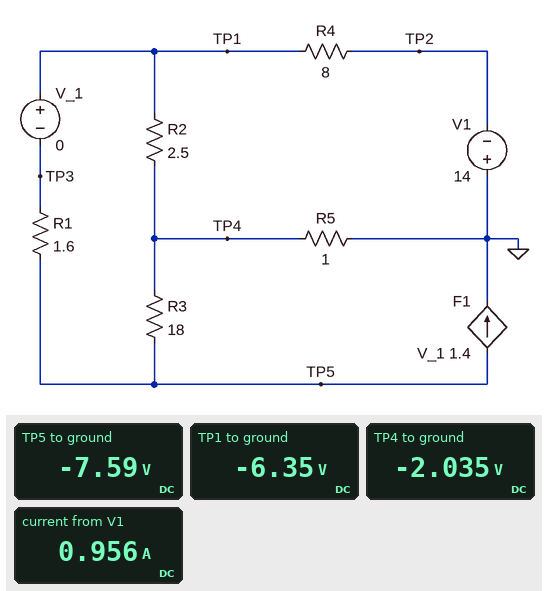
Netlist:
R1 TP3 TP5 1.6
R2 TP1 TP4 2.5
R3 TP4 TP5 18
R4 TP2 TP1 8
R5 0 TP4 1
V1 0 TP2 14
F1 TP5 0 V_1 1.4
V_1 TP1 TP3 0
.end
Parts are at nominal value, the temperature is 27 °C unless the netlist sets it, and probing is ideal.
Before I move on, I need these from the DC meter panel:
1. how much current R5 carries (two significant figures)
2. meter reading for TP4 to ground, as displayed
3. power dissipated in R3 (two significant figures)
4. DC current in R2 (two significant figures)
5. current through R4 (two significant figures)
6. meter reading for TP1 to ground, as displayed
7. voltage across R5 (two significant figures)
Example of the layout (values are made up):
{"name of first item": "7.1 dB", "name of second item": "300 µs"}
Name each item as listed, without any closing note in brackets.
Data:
{"how much current R5 carries": "2.0 A", "meter reading for TP4 to ground, as displayed": "-2.035 V", "power dissipated in R3": "1.7 W", "DC current in R2": "1.7 A", "current through R4": "960 mA", "meter reading for TP1 to ground, as displayed": "-6.35 V", "voltage across R5": "2.0 V"}
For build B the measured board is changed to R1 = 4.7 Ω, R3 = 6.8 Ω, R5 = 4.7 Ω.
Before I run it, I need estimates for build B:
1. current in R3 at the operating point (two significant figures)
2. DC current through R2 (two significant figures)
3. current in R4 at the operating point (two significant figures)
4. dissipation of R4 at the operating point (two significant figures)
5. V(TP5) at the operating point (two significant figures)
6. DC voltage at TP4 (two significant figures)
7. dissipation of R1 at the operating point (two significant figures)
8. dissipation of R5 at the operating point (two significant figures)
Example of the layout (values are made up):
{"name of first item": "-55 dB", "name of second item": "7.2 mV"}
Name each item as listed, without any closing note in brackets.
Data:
{"current in R3 at the operating point": "310 mA", "DC current through R2": "610 mA", "current in R4 at the operating point": "1.4 A", "dissipation of R4 at the operating point": "15 W", "V(TP5) at the operating point": "680 mV", "DC voltage at TP4": "-1.4 V", "dissipation of R1 at the operating point": "2.8 W", "dissipation of R5 at the operating point": "430 mW"}
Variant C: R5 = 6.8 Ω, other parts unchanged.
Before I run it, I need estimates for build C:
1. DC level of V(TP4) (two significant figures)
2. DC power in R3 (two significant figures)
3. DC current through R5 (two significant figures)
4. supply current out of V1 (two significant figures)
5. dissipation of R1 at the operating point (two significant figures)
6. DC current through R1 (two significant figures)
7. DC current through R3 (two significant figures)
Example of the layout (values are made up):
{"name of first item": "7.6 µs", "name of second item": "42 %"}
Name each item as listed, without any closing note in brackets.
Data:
{"DC level of V(TP4)": "-7.5 V", "DC power in R3": "500 mW", "DC current through R5": "1.1 A", "supply current out of V1": "520 mA", "dissipation of R1 at the operating point": "280 mW", "DC current through R1": "420 mA", "DC current through R3": "170 mA"}
